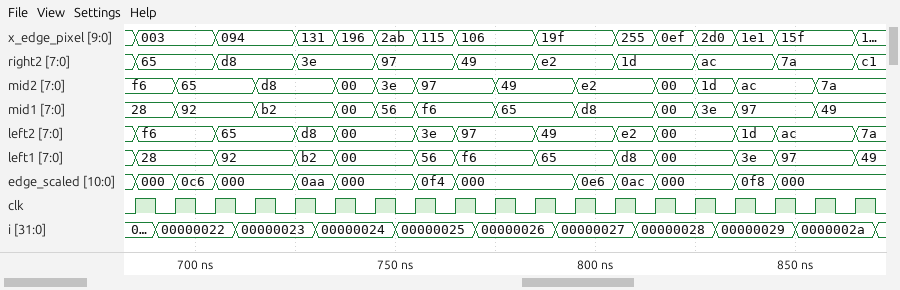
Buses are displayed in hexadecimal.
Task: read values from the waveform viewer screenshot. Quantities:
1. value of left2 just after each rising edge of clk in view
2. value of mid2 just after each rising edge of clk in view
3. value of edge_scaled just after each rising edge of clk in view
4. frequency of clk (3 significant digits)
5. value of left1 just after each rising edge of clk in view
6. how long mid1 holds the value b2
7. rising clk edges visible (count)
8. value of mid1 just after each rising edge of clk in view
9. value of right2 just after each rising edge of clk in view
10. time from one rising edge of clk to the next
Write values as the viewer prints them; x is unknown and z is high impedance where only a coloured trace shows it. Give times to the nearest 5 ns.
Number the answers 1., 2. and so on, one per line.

1. f6, f6, 65, 65, d8, 00, 00, 3e, 97, 97, 49, 49, e2, 00, 00, 1d, ac, ac, 7a
2. f6, 65, 65, d8, d8, 00, 3e, 97, 97, 49, 49, e2, e2, 00, 1d, ac, ac, 7a, 7a
3. 000, 0c6, 000, 000, 0aa, 000, 000, 0f4, 000, 000, 000, 0e6, 0ac, 000, 000, 0f8, 000, 000, 000
4. 100 MHz
5. 28, 28, 92, 92, b2, 00, 00, 56, f6, f6, 65, 65, d8, 00, 00, 3e, 97, 97, 49
6. 20 ns
7. 19
8. 28, 92, 92, b2, b2, 00, 56, f6, f6, 65, 65, d8, d8, 00, 3e, 97, 97, 49, 49
9. 65, 65, d8, d8, 3e, 3e, 97, 97, 49, 49, e2, e2, 1d, 1d, ac, ac, 7a, 7a, c1
10. 10 ns
